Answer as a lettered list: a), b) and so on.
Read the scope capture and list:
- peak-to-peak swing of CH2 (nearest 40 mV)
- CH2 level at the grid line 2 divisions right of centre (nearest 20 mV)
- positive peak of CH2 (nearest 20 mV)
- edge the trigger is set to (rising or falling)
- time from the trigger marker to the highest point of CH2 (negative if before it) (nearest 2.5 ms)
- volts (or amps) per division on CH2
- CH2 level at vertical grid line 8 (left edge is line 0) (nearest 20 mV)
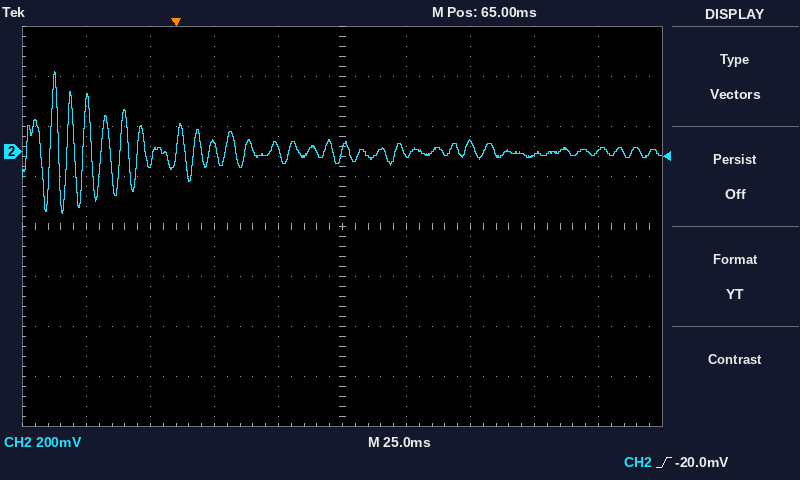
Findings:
a) 560 mV
b) 40 mV
c) 320 mV
d) rising
e) -47.5 ms
f) 200 mV
g) -20 mV
